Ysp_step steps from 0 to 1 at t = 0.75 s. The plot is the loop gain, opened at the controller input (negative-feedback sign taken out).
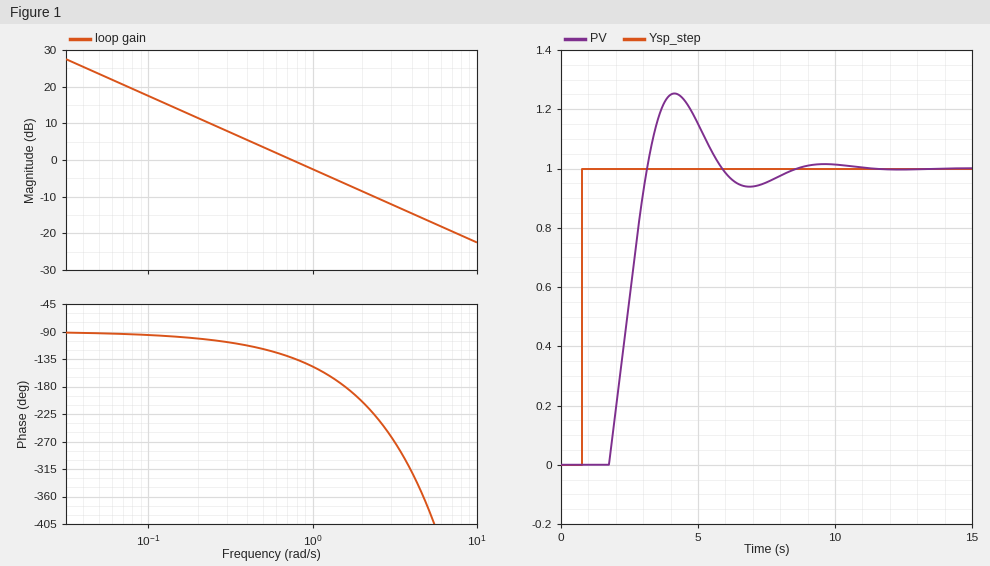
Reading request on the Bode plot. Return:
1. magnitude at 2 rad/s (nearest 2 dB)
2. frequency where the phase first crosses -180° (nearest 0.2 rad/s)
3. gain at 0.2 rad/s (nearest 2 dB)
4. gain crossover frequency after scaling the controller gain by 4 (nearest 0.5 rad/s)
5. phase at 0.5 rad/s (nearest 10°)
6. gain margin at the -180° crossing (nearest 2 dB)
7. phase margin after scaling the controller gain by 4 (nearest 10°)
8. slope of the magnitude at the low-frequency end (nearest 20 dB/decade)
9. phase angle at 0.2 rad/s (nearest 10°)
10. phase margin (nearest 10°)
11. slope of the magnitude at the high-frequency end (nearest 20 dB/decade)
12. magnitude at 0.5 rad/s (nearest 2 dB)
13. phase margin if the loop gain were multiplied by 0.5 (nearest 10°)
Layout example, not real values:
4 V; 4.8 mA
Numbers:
-8 dB; 1.6 rad/s; 12 dB; 3.0 rad/s; -120°; 6 dB; -80°; -20 dB/decade; -100°; 50°; -20 dB/decade; 4 dB; 70°
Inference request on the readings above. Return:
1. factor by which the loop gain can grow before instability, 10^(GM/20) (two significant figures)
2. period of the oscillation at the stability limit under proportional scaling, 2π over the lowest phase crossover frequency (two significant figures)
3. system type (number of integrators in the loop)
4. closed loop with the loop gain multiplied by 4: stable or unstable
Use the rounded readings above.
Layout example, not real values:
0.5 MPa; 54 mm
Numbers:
2.0; 3.9 s; 1; unstable
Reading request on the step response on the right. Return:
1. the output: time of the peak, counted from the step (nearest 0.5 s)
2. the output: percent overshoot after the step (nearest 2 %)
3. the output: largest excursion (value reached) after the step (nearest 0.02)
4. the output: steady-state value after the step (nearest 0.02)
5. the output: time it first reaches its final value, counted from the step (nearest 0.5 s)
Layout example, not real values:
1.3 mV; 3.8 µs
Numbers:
3.5 s; 26 %; 1.26; 1.00; 2.5 s
